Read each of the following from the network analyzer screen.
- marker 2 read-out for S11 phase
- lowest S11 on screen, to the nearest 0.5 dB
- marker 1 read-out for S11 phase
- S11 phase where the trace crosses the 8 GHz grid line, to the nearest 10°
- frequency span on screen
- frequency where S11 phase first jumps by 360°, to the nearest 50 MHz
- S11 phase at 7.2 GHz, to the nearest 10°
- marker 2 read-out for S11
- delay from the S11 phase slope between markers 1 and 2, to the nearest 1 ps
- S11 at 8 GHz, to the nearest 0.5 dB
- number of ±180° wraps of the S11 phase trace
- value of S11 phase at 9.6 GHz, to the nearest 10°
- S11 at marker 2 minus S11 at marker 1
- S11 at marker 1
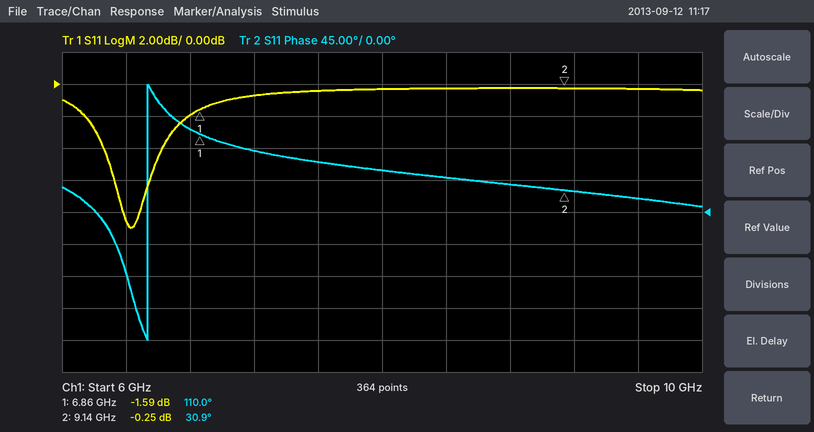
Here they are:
30.9°
-9.0 dB
110.0°
60°
4 GHz
6.55 GHz
90°
-0.25 dB
96 ps
-0.5 dB
1
20°
1.34 dB
-1.59 dB
